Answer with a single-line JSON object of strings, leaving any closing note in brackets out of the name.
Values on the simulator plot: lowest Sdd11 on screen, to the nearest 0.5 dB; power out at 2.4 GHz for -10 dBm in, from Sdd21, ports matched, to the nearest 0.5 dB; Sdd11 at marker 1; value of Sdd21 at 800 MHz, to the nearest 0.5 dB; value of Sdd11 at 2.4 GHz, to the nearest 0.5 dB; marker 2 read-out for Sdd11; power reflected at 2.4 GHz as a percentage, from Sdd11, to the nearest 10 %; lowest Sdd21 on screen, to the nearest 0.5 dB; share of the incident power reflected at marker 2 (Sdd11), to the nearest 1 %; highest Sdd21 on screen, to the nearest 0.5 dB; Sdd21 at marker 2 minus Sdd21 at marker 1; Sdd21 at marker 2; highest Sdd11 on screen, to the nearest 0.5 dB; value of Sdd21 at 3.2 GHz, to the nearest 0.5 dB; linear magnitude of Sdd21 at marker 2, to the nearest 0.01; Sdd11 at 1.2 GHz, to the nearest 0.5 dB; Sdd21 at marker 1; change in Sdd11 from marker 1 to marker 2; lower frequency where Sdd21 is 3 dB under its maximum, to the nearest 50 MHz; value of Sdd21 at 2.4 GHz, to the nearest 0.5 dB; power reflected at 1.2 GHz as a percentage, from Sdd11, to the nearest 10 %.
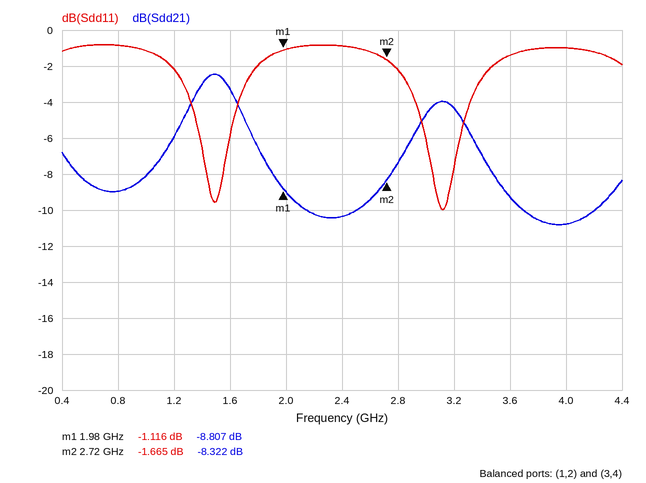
{"lowest Sdd11 on screen, to the nearest 0.5 dB": "-10.0 dB", "power out at 2.4 GHz for -10 dBm in, from Sdd21, ports matched, to the nearest 0.5 dB": "-20.5 dBm", "Sdd11 at marker 1": "-1.116 dB", "value of Sdd21 at 800 MHz, to the nearest 0.5 dB": "-9.0 dB", "value of Sdd11 at 2.4 GHz, to the nearest 0.5 dB": "-1.0 dB", "marker 2 read-out for Sdd11": "-1.665 dB", "power reflected at 2.4 GHz as a percentage, from Sdd11, to the nearest 10 %": "80 %", "lowest Sdd21 on screen, to the nearest 0.5 dB": "-11.0 dB", "share of the incident power reflected at marker 2 (Sdd11), to the nearest 1 %": "68 %", "highest Sdd21 on screen, to the nearest 0.5 dB": "-2.5 dB", "Sdd21 at marker 2 minus Sdd21 at marker 1": "0.485 dB", "Sdd21 at marker 2": "-8.322 dB", "highest Sdd11 on screen, to the nearest 0.5 dB": "-1.0 dB", "value of Sdd21 at 3.2 GHz, to the nearest 0.5 dB": "-4.5 dB", "linear magnitude of Sdd21 at marker 2, to the nearest 0.01": "0.38", "Sdd11 at 1.2 GHz, to the nearest 0.5 dB": "-2.0 dB", "Sdd21 at marker 1": "-8.807 dB", "change in Sdd11 from marker 1 to marker 2": "-0.549 dB", "lower frequency where Sdd21 is 3 dB under its maximum, to the nearest 50 MHz": "1.25 GHz", "value of Sdd21 at 2.4 GHz, to the nearest 0.5 dB": "-10.5 dB", "power reflected at 1.2 GHz as a percentage, from Sdd11, to the nearest 10 %": "60 %"}
